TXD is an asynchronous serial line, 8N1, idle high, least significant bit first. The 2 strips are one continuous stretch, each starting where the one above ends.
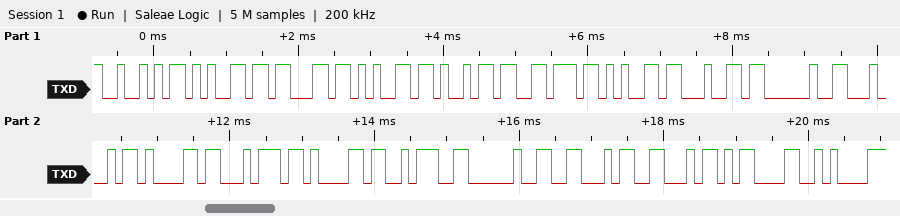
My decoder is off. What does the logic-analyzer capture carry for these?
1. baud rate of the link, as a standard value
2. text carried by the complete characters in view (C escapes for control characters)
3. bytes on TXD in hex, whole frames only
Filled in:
9600 baud
"Received Data: FF\r\n"
52 65 63 65 69 76 65 64 20 44 61 74 61 3A 20 46 46 0D 0A
